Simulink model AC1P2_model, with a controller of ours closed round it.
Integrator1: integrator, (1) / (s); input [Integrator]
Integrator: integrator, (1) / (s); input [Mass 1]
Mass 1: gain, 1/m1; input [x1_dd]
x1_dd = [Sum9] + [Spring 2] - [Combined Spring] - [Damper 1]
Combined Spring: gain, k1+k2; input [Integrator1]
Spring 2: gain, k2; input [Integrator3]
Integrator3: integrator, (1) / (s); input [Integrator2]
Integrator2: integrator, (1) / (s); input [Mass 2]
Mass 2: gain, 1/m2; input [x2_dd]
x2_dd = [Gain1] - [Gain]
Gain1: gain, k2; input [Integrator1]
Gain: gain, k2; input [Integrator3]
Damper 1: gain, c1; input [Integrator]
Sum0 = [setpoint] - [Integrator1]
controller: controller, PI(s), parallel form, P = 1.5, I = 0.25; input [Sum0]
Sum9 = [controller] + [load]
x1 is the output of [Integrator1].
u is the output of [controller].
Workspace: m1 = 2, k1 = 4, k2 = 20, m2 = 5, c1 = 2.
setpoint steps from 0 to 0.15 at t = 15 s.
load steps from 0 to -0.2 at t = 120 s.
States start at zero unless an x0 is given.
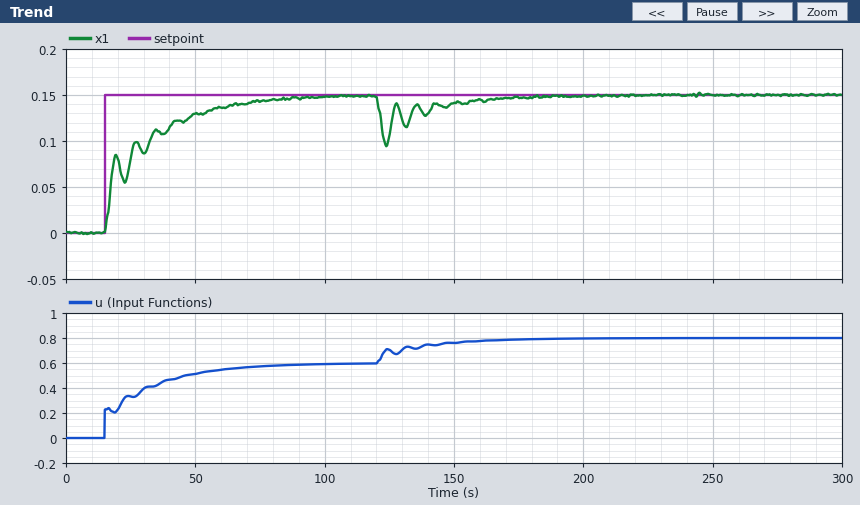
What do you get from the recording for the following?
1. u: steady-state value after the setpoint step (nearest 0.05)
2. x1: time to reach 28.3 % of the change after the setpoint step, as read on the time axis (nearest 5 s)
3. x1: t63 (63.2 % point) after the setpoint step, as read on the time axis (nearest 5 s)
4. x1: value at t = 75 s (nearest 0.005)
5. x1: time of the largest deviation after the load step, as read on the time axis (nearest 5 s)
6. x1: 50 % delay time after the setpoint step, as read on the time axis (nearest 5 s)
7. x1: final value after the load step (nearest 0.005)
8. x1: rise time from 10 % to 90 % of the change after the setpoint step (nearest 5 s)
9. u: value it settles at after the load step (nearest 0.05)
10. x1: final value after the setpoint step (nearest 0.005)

0.60
15 s
25 s
0.145
125 s
20 s
0.150
40 s
0.80
0.150
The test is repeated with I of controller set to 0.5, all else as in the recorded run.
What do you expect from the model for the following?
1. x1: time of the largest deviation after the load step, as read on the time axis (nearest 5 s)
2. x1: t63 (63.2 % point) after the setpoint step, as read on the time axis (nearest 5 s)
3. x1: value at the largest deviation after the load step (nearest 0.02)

125 s
20 s
0.10
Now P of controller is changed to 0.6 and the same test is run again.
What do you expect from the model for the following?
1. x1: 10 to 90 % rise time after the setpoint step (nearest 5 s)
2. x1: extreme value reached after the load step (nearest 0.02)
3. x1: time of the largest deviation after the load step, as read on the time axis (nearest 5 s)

35 s
0.08
125 s
